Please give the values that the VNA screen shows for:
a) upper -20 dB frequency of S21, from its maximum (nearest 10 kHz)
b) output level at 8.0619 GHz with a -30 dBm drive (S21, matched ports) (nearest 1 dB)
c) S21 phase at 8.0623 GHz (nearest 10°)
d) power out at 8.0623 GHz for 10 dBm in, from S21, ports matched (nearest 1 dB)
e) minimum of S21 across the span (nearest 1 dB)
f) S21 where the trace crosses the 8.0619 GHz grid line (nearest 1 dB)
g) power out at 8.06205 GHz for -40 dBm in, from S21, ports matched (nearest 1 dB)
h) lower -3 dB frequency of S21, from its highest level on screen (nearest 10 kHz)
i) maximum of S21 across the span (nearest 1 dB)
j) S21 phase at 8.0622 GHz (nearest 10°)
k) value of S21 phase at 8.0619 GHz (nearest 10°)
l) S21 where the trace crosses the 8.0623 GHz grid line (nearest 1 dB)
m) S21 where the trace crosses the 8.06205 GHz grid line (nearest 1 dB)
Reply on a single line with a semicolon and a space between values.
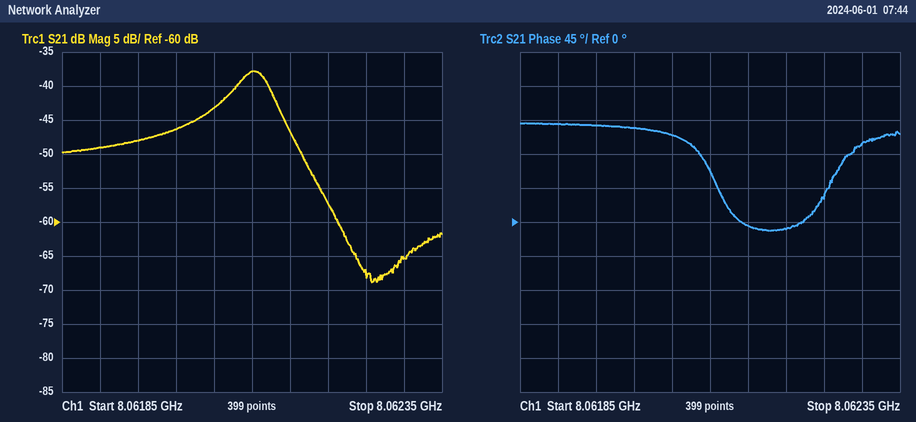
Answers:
8.06220 GHz; -79 dBm; 100°; -55 dBm; -69 dB; -49 dB; -83 dBm; 8.06207 GHz; -38 dB; -10°; 130°; -65 dB; -43 dB
